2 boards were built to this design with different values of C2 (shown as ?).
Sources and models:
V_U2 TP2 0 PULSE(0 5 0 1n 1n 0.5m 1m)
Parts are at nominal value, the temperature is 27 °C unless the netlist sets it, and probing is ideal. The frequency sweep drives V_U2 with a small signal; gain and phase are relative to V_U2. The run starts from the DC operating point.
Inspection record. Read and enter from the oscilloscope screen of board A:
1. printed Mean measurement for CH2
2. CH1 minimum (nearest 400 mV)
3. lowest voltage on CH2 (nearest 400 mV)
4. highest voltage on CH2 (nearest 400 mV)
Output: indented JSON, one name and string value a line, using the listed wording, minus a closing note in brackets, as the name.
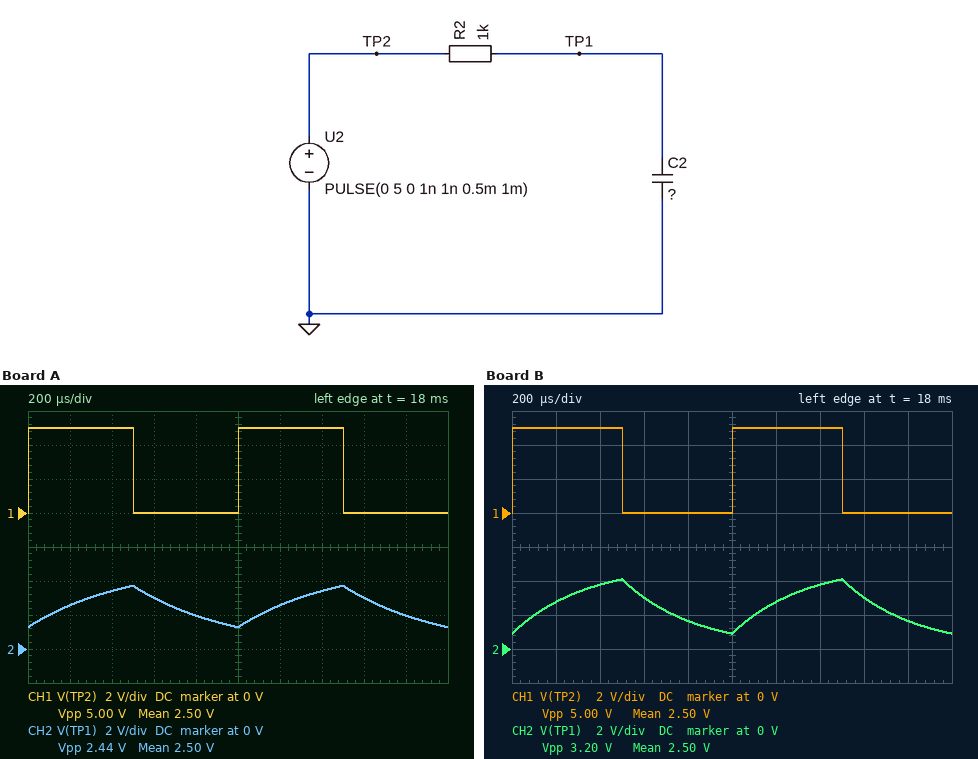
{
  "printed Mean measurement for CH2": "2.50 V",
  "CH1 minimum": "0 V",
  "lowest voltage on CH2": "1.2 V",
  "highest voltage on CH2": "3.6 V"
}
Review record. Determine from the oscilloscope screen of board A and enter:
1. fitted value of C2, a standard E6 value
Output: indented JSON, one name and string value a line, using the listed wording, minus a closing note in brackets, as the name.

{
  "fitted value of C2, a standard E6 value": "470 nF"
}
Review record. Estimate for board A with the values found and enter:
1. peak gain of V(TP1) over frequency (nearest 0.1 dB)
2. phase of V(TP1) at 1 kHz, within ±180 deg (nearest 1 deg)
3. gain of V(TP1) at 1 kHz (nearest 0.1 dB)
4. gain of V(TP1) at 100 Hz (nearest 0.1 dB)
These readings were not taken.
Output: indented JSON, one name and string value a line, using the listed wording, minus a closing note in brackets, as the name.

{
  "peak gain of V(TP1) over frequency": "0 dB",
  "phase of V(TP1) at 1 kHz, within ±180 deg": "-71 deg",
  "gain of V(TP1) at 1 kHz": "-9.9 dB",
  "gain of V(TP1) at 100 Hz": "-0.4 dB"
}
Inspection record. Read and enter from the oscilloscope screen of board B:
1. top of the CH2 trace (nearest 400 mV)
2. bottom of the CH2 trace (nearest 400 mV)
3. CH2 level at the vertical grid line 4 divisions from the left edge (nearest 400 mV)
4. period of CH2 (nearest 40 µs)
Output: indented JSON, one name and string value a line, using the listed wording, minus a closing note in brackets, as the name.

{
  "top of the CH2 trace": "4.0 V",
  "bottom of the CH2 trace": "800 mV",
  "CH2 level at the vertical grid line 4 divisions from the left edge": "1.6 V",
  "period of CH2": "1.00 ms"
}
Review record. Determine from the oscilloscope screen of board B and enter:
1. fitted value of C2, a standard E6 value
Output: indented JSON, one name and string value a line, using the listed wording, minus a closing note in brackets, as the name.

{
  "fitted value of C2, a standard E6 value": "330 nF"
}
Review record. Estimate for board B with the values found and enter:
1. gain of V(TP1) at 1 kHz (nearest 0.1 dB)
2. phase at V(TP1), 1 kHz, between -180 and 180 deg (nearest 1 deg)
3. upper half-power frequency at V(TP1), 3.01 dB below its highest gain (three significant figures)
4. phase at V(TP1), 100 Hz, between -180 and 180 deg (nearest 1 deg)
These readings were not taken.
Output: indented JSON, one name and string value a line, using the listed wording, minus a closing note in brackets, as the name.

{
  "gain of V(TP1) at 1 kHz": "-7.2 dB",
  "phase at V(TP1), 1 kHz, between -180 and 180 deg": "-64 deg",
  "upper half-power frequency at V(TP1), 3.01 dB below its highest gain": "482 Hz",
  "phase at V(TP1), 100 Hz, between -180 and 180 deg": "-12 deg"
}
